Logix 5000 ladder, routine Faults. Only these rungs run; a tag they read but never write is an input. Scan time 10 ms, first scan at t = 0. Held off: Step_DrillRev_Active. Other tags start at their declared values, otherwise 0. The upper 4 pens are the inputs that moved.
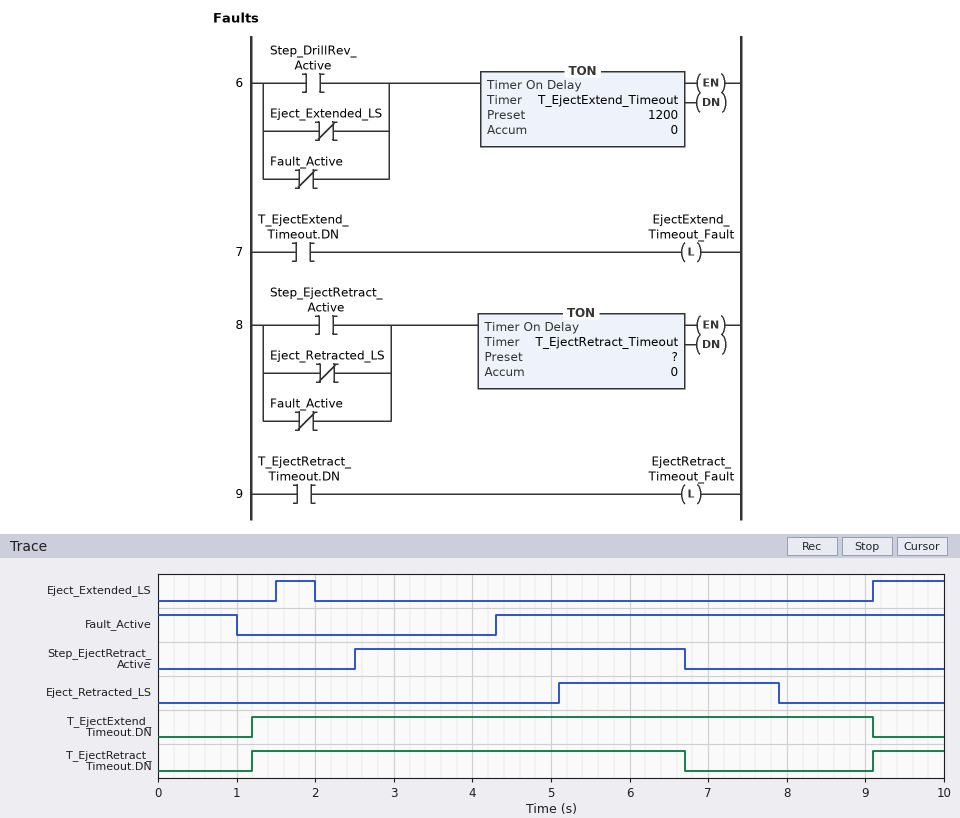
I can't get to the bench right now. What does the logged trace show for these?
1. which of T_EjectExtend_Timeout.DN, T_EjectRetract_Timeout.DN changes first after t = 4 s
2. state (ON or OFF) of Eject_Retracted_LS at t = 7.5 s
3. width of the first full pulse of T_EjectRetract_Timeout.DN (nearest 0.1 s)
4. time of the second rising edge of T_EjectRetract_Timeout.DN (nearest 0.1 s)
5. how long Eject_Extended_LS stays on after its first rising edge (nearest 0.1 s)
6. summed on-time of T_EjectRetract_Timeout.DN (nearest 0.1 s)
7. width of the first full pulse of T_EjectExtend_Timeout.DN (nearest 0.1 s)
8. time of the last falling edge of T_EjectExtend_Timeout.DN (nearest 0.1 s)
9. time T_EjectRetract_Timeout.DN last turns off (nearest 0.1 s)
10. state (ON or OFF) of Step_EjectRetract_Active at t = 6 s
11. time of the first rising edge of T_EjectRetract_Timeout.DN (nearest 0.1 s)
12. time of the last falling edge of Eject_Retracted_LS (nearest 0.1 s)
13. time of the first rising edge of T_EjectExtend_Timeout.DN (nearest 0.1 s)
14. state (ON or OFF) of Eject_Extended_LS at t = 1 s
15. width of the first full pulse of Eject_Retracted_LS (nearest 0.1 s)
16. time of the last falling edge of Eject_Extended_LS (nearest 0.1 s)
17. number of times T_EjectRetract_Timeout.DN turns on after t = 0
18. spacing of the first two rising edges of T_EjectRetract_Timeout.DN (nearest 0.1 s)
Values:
T_EjectRetract_Timeout.DN
ON
5.5 s
9.1 s
0.5 s
6.4 s
7.9 s
9.1 s
6.7 s
ON
1.2 s
7.9 s
1.2 s
OFF
2.8 s
2.0 s
2
7.9 s
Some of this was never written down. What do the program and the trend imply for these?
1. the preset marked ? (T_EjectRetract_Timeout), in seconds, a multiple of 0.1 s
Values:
1.2 s
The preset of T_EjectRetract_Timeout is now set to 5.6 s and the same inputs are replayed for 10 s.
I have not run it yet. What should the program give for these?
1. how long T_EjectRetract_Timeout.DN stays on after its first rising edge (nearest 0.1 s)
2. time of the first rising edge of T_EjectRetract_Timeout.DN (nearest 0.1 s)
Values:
1.1 s
5.6 s
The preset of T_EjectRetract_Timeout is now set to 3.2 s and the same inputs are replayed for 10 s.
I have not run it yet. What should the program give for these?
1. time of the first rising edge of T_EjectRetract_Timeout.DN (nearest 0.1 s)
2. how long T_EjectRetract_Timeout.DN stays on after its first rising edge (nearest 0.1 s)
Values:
3.2 s
3.5 s
